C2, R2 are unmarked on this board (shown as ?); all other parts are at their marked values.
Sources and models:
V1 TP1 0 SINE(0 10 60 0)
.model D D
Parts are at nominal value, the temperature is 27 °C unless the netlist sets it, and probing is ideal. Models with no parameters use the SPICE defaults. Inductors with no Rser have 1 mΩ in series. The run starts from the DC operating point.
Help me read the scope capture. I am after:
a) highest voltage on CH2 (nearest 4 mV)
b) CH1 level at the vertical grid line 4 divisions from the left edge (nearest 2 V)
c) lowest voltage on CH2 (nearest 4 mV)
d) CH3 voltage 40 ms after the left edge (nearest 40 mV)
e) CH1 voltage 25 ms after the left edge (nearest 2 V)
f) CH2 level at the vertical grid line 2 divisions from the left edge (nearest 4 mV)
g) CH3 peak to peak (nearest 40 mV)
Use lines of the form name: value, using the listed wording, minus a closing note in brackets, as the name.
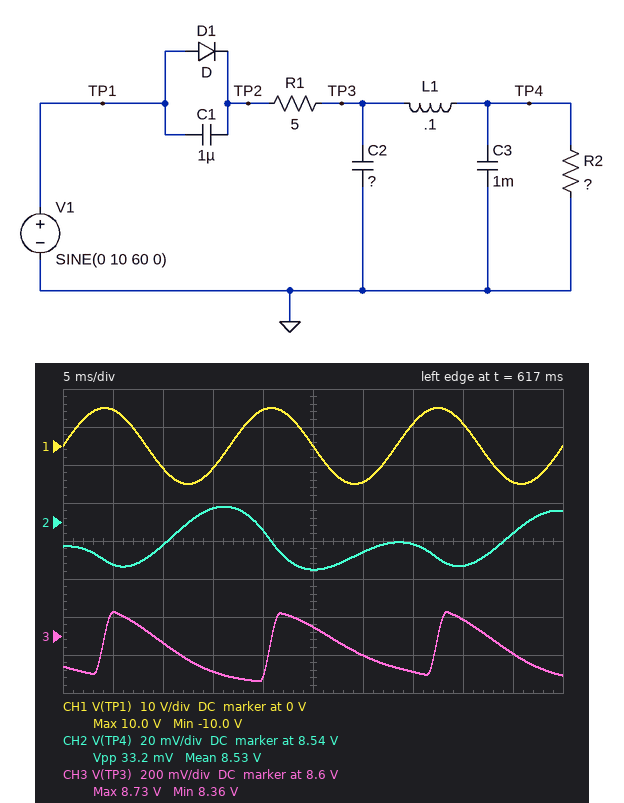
highest voltage on CH2: 8.548 V
CH1 level at the vertical grid line 4 divisions from the left edge: 10 V
lowest voltage on CH2: 8.516 V
CH3 voltage 40 ms after the left edge: 8.68 V
CH1 voltage 25 ms after the left edge: 0 V
CH2 level at the vertical grid line 2 divisions from the left edge: 8.528 V
CH3 peak to peak: 360 mV
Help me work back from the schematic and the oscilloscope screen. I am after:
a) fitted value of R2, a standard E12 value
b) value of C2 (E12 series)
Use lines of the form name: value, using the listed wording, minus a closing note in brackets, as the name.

fitted value of R2, a standard E12 value: 820 Ω
value of C2: 470 µF
